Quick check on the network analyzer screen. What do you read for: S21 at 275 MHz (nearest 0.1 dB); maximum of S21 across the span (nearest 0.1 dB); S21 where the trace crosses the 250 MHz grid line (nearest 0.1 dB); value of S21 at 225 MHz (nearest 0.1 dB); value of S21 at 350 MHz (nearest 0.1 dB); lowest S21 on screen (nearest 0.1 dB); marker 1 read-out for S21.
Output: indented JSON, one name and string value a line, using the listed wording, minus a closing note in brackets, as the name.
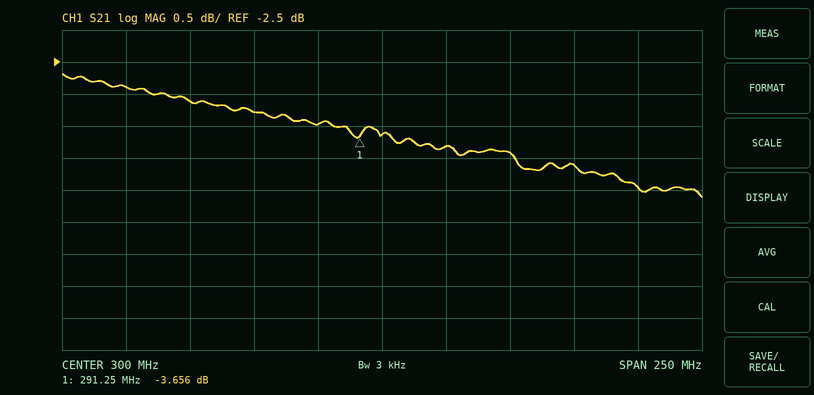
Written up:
{
  "S21 at 275 MHz": "-3.5 dB",
  "maximum of S21 across the span": "-2.7 dB",
  "S21 where the trace crosses the 250 MHz grid line": "-3.3 dB",
  "value of S21 at 225 MHz": "-3.1 dB",
  "value of S21 at 350 MHz": "-3.9 dB",
  "lowest S21 on screen": "-4.6 dB",
  "marker 1 read-out for S21": "-3.656 dB"
}
